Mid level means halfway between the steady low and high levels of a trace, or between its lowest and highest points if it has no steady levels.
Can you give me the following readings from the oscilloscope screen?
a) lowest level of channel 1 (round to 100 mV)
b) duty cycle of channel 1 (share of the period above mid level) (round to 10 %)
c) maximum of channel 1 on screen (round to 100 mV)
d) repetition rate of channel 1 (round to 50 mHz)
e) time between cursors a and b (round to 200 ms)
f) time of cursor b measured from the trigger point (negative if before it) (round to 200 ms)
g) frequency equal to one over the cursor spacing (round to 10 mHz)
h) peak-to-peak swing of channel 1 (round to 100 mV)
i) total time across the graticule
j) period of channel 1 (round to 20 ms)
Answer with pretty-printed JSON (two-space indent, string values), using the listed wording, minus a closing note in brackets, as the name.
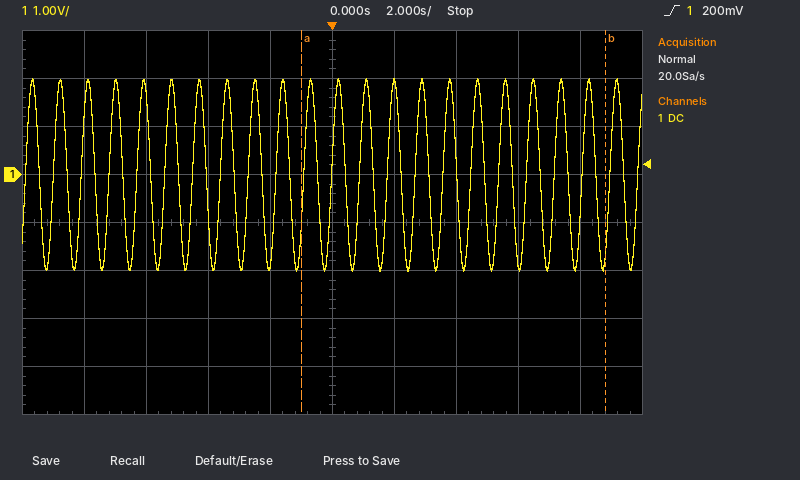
{
  "lowest level of channel 1": "-2.0 V",
  "duty cycle of channel 1 (share of the period above mid level)": "50 %",
  "maximum of channel 1 on screen": "2.0 V",
  "repetition rate of channel 1": "1.10 Hz",
  "time between cursors a and b": "9.8 s",
  "time of cursor b measured from the trigger point (negative if before it)": "+8.8 s",
  "frequency equal to one over the cursor spacing": "100 mHz",
  "peak-to-peak swing of channel 1": "4.0 V",
  "total time across the graticule": "20 s",
  "period of channel 1": "900 ms"
}
